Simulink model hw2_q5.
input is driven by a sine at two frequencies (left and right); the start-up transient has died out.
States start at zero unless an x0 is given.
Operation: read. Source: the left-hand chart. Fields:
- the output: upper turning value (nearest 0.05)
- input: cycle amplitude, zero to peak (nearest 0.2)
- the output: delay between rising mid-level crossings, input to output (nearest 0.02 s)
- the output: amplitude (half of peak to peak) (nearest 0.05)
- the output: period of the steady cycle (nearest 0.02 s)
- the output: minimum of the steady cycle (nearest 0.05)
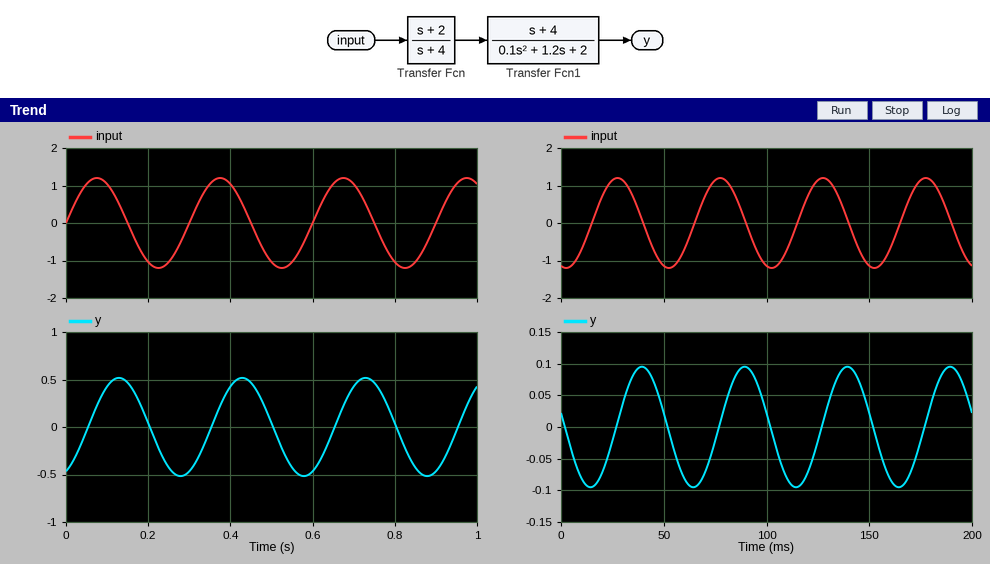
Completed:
0.50
1.2
0.06 s
0.50
0.30 s
-0.50
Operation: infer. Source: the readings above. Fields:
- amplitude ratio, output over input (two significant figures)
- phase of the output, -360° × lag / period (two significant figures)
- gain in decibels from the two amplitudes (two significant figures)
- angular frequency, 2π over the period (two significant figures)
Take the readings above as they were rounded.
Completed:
0.42
-72°
-7.6 dB
21 rad/s
